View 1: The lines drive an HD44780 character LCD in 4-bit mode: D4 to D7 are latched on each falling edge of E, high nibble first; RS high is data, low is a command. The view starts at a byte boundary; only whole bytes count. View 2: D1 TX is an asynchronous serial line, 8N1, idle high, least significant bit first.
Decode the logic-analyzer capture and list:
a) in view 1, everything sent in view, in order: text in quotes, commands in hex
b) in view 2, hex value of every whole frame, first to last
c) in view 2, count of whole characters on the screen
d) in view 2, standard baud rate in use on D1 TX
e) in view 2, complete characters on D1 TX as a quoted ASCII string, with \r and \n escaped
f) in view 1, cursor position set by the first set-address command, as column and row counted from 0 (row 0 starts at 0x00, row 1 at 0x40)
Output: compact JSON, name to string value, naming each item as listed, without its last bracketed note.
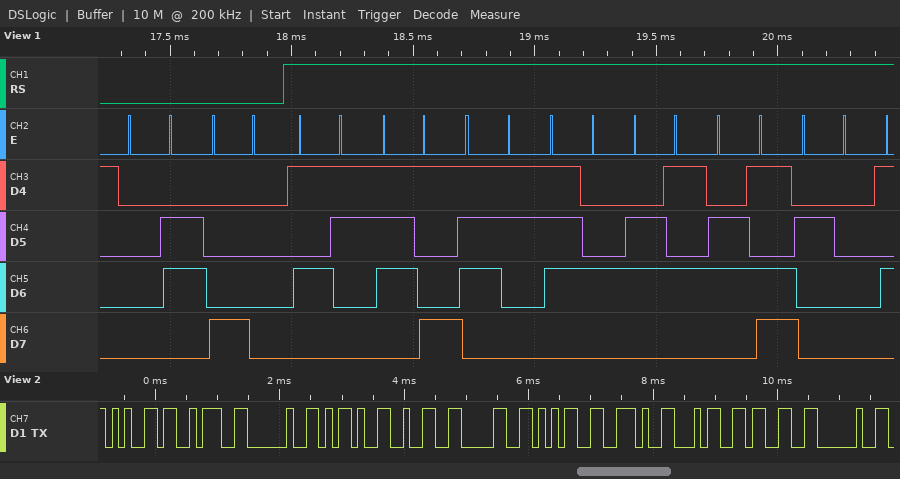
{"in view 1, everything sent in view, in order: text in quotes, commands in hex": "0x06 0x80 \"System \"", "in view 2, hex value of every whole frame, first to last": "0x65 0x3A 0x20 0x2D 0x32 0x30 0x35 0x2E 0x34 0x33 0x20", "in view 2, count of whole characters on the screen": "11", "in view 2, standard baud rate in use on D1 TX": "9600 baud", "in view 2, complete characters on D1 TX as a quoted ASCII string, with \\r and \\n escaped": "\"e: -205.43 \"", "in view 1, cursor position set by the first set-address command, as column and row counted from 0": "column 0, row 0"}
